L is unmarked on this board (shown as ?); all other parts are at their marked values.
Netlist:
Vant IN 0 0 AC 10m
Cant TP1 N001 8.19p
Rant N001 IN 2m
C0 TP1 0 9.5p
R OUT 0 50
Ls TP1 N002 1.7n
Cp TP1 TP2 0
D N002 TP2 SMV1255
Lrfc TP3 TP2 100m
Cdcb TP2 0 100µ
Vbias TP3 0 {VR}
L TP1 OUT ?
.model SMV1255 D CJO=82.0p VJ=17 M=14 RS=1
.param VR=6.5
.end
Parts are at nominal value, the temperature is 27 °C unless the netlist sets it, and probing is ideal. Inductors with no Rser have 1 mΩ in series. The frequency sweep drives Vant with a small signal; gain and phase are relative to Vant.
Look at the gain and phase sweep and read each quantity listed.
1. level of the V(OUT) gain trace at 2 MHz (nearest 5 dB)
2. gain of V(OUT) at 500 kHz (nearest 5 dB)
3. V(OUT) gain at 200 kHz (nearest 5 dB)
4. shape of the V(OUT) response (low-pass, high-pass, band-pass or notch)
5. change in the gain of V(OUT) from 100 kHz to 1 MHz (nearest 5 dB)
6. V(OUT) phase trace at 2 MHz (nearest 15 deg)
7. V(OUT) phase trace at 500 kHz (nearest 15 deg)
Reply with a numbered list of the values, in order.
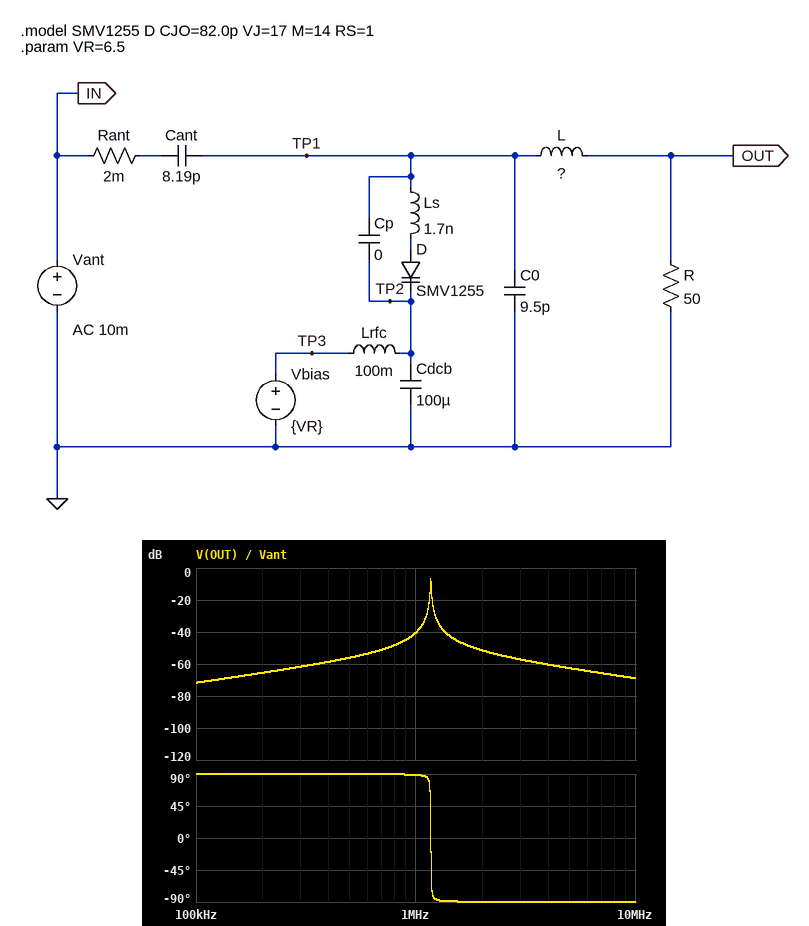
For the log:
1. -50 dB
2. -55 dB
3. -65 dB
4. band-pass
5. 30 dB
6. -90 deg
7. 90 deg
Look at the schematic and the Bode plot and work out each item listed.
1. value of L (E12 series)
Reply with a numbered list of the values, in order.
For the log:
1. 1 mH
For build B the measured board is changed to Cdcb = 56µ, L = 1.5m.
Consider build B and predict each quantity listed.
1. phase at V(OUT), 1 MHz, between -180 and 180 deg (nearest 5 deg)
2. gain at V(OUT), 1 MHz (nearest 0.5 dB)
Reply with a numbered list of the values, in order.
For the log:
1. -85 deg
2. -32.0 dB
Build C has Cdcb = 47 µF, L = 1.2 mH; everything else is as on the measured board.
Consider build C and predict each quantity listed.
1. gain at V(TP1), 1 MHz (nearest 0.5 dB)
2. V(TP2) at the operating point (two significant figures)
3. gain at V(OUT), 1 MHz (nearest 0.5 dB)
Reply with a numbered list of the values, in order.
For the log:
1. 10.0 dB
2. 6.5 V
3. -33.5 dB
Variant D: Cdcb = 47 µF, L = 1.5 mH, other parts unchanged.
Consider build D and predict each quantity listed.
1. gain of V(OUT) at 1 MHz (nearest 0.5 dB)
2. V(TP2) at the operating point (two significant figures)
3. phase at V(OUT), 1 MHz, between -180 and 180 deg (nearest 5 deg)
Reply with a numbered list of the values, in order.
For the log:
1. -32.0 dB
2. 6.5 V
3. -85 deg
